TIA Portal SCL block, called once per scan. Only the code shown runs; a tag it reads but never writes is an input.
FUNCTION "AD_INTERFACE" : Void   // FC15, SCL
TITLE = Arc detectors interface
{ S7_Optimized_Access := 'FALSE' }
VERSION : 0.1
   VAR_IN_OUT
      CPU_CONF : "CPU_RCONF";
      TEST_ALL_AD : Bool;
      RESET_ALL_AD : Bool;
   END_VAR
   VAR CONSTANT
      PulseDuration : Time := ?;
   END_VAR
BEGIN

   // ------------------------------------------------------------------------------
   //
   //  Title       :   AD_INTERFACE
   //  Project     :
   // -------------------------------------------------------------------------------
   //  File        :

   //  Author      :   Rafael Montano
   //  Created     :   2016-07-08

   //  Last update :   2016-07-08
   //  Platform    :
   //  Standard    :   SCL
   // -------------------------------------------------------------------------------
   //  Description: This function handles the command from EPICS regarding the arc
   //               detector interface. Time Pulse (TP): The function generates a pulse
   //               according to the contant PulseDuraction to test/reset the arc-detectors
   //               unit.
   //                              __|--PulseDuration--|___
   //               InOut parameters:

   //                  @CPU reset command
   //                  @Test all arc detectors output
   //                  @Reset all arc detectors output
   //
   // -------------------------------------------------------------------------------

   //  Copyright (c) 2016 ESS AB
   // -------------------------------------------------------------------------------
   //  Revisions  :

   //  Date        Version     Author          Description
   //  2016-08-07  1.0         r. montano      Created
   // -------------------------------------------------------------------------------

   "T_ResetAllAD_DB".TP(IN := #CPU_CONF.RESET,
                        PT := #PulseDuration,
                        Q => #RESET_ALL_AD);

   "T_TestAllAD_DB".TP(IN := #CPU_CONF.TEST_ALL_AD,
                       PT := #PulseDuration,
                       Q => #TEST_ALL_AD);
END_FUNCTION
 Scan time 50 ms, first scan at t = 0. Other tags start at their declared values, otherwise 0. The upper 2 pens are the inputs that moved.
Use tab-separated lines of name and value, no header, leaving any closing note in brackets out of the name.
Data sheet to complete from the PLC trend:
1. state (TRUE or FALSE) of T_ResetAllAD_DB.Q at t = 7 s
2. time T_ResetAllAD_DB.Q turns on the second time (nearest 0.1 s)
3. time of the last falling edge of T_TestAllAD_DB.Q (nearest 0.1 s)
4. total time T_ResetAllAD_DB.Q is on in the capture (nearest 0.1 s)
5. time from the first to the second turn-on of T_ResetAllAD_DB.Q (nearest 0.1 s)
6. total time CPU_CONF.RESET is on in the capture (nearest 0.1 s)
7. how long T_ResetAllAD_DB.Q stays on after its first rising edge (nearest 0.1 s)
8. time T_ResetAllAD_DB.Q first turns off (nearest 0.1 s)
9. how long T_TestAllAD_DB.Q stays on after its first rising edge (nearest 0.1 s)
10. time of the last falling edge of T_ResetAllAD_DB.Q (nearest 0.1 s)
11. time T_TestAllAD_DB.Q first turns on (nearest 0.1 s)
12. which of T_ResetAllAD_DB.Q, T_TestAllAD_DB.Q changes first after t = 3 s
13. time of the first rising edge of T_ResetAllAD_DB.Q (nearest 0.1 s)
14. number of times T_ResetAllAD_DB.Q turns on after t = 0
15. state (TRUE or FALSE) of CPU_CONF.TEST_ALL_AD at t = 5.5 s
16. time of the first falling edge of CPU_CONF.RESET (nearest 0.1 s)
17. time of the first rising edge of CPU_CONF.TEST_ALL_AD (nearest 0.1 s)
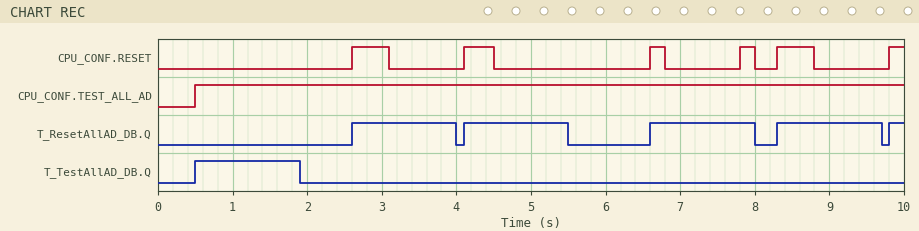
state (TRUE or FALSE) of T_ResetAllAD_DB.Q at t = 7 s	TRUE
time T_ResetAllAD_DB.Q turns on the second time	4.1 s
time of the last falling edge of T_TestAllAD_DB.Q	1.9 s
total time T_ResetAllAD_DB.Q is on in the capture	5.8 s
time from the first to the second turn-on of T_ResetAllAD_DB.Q	1.5 s
total time CPU_CONF.RESET is on in the capture	2.0 s
how long T_ResetAllAD_DB.Q stays on after its first rising edge	1.4 s
time T_ResetAllAD_DB.Q first turns off	4.0 s
how long T_TestAllAD_DB.Q stays on after its first rising edge	1.4 s
time of the last falling edge of T_ResetAllAD_DB.Q	9.7 s
time T_TestAllAD_DB.Q first turns on	0.5 s
which of T_ResetAllAD_DB.Q, T_TestAllAD_DB.Q changes first after t = 3 s	T_ResetAllAD_DB.Q
time of the first rising edge of T_ResetAllAD_DB.Q	2.6 s
number of times T_ResetAllAD_DB.Q turns on after t = 0	5
state (TRUE or FALSE) of CPU_CONF.TEST_ALL_AD at t = 5.5 s	TRUE
time of the first falling edge of CPU_CONF.RESET	3.1 s
time of the first rising edge of CPU_CONF.TEST_ALL_AD	0.5 s
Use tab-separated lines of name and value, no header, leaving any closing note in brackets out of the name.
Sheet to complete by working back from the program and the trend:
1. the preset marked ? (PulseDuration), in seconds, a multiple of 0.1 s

the preset marked ? (PulseDuration), in seconds, a multiple of 0.1 s	1.4 s
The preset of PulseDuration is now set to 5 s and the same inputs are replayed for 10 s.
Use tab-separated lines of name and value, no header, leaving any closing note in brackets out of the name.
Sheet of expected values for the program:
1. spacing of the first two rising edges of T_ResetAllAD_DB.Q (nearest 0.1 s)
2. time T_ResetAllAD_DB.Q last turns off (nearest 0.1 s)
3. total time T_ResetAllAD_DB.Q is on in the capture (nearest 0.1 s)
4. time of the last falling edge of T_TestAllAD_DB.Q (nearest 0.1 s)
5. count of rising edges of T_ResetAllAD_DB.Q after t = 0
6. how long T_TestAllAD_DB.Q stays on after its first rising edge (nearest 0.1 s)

spacing of the first two rising edges of T_ResetAllAD_DB.Q	5.2 s
time T_ResetAllAD_DB.Q last turns off	7.6 s
total time T_ResetAllAD_DB.Q is on in the capture	7.2 s
time of the last falling edge of T_TestAllAD_DB.Q	5.5 s
count of rising edges of T_ResetAllAD_DB.Q after t = 0	2
how long T_TestAllAD_DB.Q stays on after its first rising edge	5.0 s
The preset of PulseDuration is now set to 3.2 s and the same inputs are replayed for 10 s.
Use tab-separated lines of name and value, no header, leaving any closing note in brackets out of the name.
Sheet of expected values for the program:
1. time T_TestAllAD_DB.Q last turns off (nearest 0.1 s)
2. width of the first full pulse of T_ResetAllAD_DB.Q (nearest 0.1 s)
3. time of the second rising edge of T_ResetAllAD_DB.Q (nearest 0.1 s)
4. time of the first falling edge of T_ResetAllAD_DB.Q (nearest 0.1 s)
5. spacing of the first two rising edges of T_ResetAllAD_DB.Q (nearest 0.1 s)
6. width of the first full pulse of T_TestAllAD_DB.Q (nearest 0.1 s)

time T_TestAllAD_DB.Q last turns off	3.7 s
width of the first full pulse of T_ResetAllAD_DB.Q	3.2 s
time of the second rising edge of T_ResetAllAD_DB.Q	6.6 s
time of the first falling edge of T_ResetAllAD_DB.Q	5.8 s
spacing of the first two rising edges of T_ResetAllAD_DB.Q	4.0 s
width of the first full pulse of T_TestAllAD_DB.Q	3.2 s
